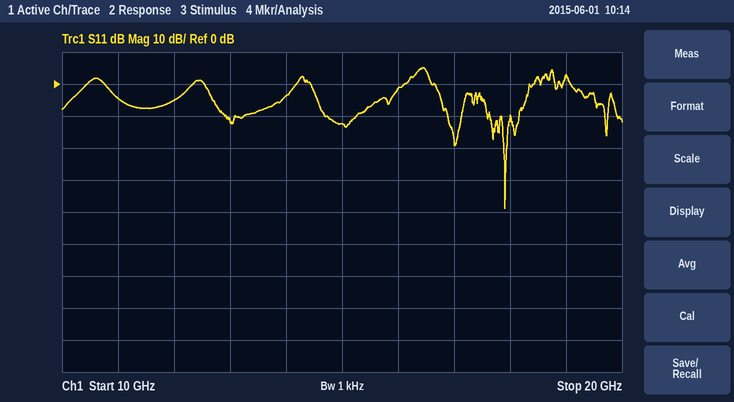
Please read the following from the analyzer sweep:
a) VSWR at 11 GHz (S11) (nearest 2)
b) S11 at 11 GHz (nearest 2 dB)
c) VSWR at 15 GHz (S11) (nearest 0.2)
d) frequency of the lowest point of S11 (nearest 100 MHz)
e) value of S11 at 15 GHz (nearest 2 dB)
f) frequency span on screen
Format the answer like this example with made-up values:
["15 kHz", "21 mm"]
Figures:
["4", "-4 dB", "1.6", "17.9 GHz", "-12 dB", "10 GHz"]
